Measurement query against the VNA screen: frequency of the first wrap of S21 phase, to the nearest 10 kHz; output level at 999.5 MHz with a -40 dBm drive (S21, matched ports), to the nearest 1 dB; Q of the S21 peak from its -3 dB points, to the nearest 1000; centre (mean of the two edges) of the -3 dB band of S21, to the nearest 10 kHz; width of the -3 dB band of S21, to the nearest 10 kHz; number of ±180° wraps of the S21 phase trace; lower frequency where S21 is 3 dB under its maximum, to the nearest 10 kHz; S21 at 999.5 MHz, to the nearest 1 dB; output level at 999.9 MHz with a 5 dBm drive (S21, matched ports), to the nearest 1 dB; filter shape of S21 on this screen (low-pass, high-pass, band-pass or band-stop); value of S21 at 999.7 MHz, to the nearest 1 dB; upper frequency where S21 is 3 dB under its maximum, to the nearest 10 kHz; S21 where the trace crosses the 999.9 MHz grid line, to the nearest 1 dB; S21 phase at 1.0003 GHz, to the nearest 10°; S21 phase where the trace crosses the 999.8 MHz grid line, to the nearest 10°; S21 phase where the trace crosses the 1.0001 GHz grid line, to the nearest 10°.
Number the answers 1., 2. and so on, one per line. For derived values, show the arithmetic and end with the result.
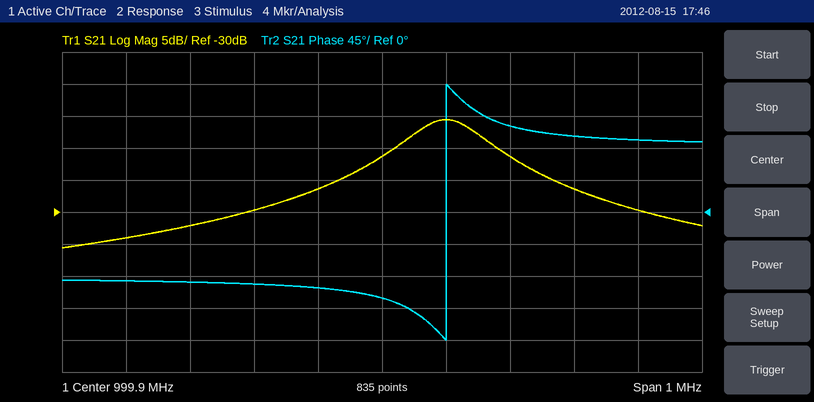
1. 1.00000 GHz
2. -40 dBm + (-34 dB) = -74 dBm
3. 1 GHz / 120 kHz ≈ 8333, so 8000 to the nearest 1000
4. 1.00000 GHz
5. 1.00006 GHz − 999.94 MHz = 120 kHz
6. 1
7. 999.94 MHz
8. -34 dB
9. 5 dBm + (-21 dB) = -16 dBm
10. band-pass
11. -30 dB
12. 1.00006 GHz
13. -21 dB
14. 100°
15. -110°
16. 120°
